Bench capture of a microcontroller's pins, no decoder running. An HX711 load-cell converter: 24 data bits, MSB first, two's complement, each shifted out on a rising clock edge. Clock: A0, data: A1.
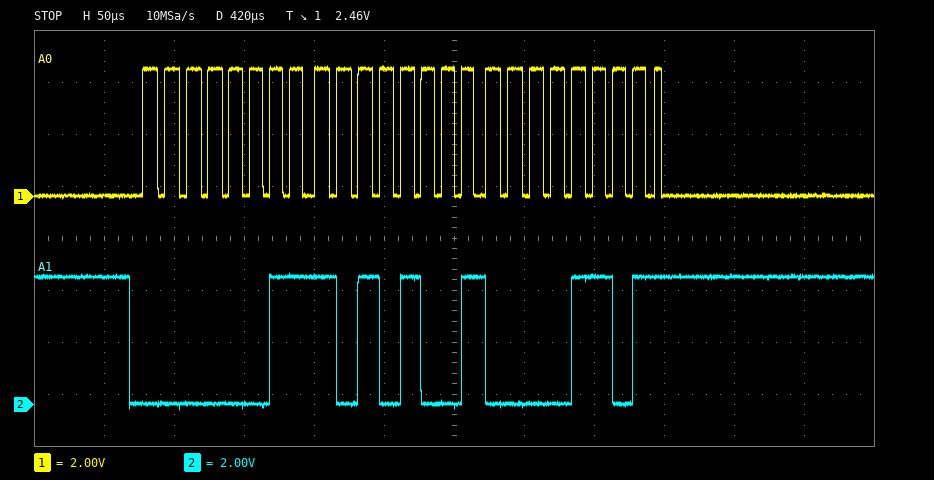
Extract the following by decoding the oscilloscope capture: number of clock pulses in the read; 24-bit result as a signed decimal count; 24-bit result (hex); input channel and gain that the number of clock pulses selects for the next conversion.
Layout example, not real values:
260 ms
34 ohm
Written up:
25
239885
0x03A90D
channel A, gain 128
